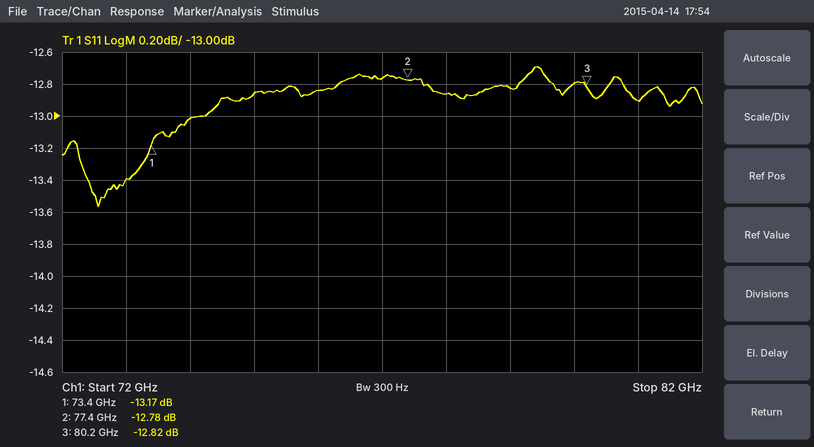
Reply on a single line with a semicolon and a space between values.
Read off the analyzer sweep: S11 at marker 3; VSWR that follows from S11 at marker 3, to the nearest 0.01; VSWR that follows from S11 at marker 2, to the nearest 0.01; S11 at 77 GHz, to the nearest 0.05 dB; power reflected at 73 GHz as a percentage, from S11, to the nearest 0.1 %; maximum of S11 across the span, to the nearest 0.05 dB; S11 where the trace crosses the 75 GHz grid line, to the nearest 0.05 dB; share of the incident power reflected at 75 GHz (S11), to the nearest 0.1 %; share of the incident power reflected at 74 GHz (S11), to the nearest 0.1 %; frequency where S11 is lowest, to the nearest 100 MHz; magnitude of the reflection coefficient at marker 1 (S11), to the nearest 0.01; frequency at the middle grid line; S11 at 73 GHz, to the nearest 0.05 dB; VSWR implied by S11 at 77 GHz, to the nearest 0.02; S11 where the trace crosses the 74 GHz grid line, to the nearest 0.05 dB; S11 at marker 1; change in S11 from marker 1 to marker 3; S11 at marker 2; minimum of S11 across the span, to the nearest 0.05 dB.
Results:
-12.82 dB; 1.59; 1.60; -12.75 dB; 4.6 %; -12.70 dB; -12.85 dB; 5.2 %; 5.0 %; 72.6 GHz; 0.22; 77 GHz; -13.40 dB; 1.60; -13.00 dB; -13.17 dB; 0.35 dB; -12.78 dB; -13.55 dB
